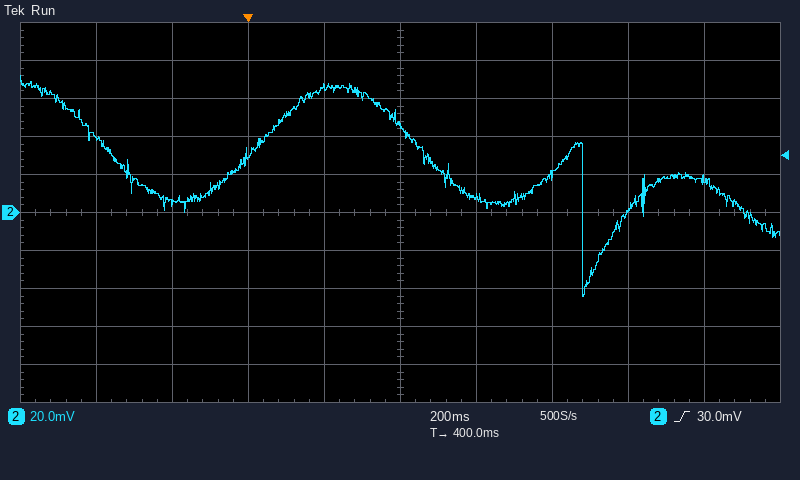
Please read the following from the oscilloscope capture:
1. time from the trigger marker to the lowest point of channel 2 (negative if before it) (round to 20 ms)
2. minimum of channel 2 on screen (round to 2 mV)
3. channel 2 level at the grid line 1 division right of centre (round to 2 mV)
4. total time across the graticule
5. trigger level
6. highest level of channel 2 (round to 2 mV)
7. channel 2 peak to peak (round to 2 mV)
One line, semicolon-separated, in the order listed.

+880 ms; -44 mV; 8 mV; 2 s; 30.0 mV; 72 mV; 116 mV
